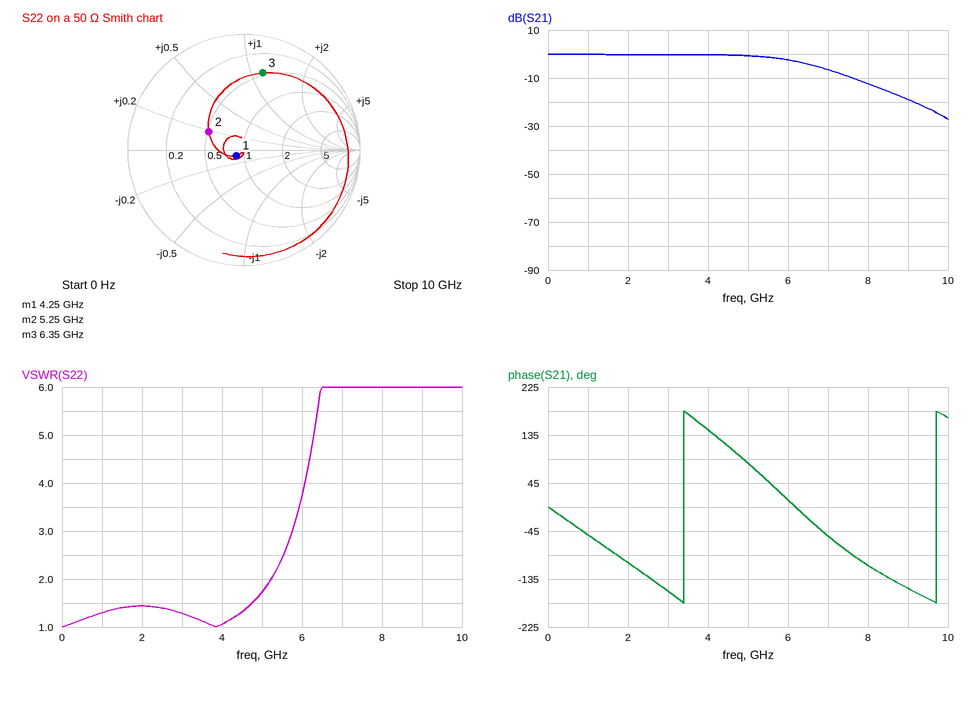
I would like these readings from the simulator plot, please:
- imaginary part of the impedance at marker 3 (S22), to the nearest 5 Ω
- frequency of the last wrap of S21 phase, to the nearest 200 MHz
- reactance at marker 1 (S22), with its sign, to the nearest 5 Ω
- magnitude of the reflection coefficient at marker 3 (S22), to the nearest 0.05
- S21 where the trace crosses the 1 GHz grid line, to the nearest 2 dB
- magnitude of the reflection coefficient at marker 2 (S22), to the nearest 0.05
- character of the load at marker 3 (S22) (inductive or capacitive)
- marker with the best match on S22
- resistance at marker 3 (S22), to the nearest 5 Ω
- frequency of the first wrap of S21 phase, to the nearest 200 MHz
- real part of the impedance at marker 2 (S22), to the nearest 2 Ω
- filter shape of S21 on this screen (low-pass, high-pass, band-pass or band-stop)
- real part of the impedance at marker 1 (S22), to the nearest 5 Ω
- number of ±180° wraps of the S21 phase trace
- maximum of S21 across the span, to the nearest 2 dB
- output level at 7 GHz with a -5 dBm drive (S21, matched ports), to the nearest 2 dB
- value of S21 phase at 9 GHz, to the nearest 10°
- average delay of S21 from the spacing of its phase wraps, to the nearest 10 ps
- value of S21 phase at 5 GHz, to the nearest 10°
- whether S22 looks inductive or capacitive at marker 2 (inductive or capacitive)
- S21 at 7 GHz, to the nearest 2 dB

+60 Ω
9.8 GHz
-5 Ω
0.70
0 dB
0.35
inductive
marker 1
25 Ω
3.4 GHz
26 Ω
low-pass
45 Ω
2
0 dB
-12 dBm
-150°
160 ps
80°
inductive
-6 dB
